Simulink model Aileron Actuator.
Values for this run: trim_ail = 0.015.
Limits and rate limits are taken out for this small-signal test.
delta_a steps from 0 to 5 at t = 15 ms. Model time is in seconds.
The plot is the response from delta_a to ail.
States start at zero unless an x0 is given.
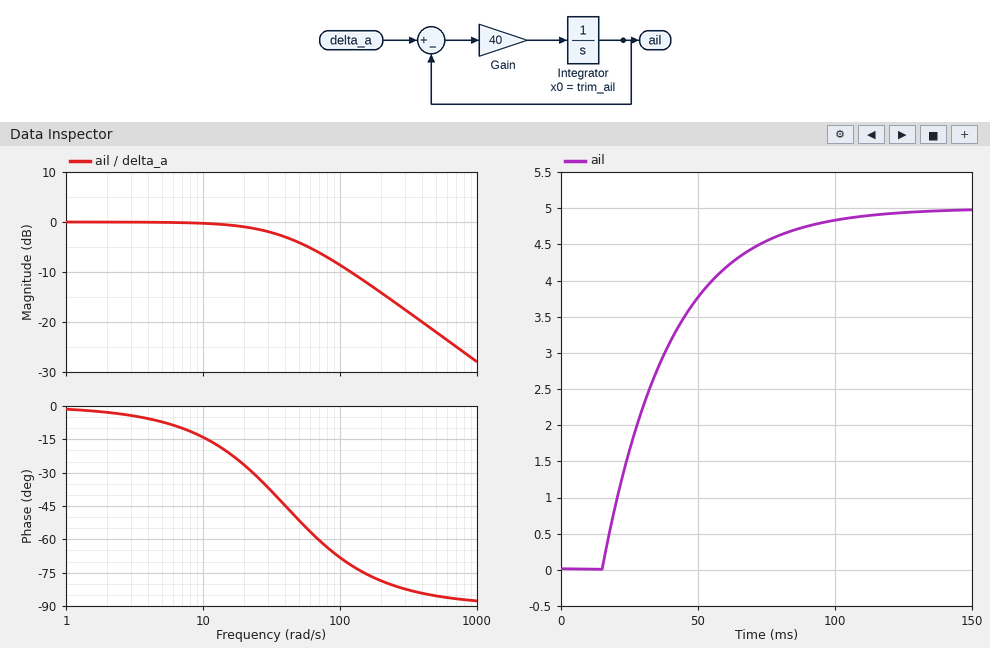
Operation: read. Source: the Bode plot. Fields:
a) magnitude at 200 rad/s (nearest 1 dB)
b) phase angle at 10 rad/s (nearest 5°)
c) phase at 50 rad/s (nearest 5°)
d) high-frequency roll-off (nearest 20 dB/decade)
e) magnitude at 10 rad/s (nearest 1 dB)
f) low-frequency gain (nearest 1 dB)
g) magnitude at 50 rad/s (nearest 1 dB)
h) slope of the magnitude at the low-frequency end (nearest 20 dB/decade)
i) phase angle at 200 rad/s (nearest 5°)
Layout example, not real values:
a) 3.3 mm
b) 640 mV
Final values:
a) -14 dB
b) -15°
c) -50°
d) -20 dB/decade
e) 0 dB
f) 0 dB
g) -4 dB
h) 0 dB/decade
i) -80°
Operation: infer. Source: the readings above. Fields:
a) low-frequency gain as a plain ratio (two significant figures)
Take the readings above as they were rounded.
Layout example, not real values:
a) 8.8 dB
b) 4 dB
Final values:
a) 1.0
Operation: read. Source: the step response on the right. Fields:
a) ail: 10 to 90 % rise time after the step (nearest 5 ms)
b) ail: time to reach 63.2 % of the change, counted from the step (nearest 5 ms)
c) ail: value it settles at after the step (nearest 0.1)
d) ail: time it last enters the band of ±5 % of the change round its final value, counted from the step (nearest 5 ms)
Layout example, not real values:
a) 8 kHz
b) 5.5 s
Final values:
a) 55 ms
b) 25 ms
c) 5.0
d) 75 ms
